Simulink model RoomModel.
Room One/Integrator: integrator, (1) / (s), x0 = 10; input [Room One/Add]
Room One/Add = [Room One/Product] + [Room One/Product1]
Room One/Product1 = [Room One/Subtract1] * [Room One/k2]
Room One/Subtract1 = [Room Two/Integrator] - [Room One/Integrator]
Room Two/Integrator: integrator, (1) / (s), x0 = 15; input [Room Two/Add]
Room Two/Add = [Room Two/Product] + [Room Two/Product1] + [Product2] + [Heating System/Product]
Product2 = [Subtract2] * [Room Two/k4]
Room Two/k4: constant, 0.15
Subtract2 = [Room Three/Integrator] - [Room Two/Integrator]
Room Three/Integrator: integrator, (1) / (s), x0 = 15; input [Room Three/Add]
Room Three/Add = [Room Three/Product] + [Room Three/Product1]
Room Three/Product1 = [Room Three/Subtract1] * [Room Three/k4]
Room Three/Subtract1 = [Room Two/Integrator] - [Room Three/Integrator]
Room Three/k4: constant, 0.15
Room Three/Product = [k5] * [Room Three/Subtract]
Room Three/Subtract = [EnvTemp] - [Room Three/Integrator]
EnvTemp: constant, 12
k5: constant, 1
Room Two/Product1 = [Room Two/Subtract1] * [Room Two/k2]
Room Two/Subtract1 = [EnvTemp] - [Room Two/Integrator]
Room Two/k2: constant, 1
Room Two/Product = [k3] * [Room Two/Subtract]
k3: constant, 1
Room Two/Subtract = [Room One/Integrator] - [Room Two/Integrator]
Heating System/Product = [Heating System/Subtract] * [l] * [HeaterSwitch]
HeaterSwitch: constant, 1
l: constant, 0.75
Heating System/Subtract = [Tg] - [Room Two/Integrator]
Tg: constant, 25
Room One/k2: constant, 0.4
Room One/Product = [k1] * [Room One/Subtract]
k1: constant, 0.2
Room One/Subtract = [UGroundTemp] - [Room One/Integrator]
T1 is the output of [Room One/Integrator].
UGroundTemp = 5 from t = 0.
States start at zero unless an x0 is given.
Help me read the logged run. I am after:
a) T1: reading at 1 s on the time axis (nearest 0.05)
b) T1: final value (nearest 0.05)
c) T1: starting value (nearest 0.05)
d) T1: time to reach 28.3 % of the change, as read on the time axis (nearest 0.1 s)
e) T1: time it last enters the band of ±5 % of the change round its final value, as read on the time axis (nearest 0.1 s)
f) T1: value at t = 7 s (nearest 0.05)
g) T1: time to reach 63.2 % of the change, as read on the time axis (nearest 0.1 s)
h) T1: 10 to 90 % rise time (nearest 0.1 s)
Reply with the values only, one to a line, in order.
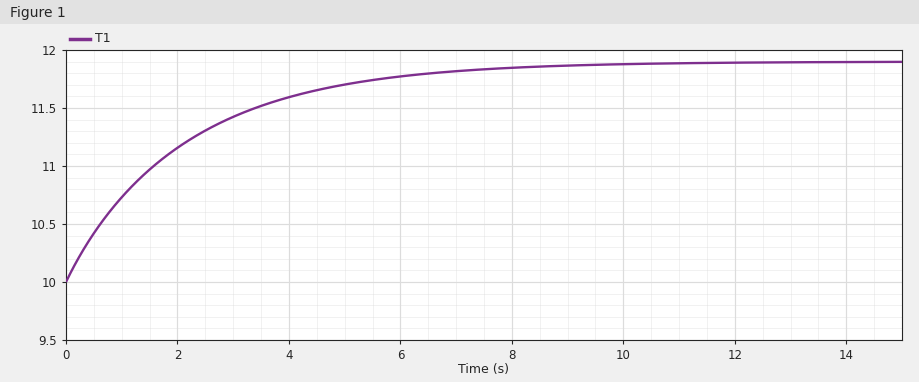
10.75
11.90
10.00
0.7 s
6.7 s
11.80
2.1 s
4.9 s
